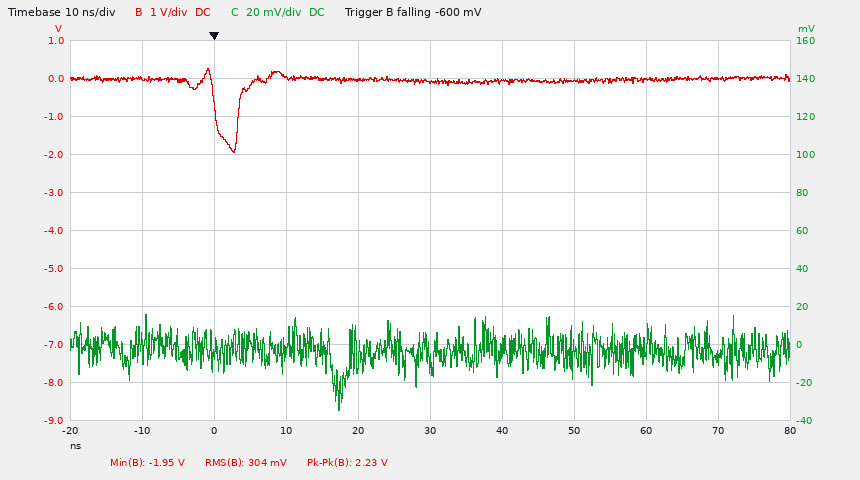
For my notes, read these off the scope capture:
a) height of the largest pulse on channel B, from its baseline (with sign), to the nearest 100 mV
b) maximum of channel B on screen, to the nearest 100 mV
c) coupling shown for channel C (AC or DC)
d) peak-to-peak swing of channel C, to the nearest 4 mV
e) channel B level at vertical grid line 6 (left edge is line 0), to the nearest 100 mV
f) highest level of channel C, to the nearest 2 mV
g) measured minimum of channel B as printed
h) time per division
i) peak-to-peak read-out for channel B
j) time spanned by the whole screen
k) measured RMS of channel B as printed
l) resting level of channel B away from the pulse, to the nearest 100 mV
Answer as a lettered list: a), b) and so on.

a) -1.9 V
b) 300 mV
c) DC
d) 52 mV
e) -100 mV
f) 16 mV
g) -1.95 V
h) 10 ns
i) 2.23 V
j) 100 ns
k) 304 mV
l) 0.0 V
